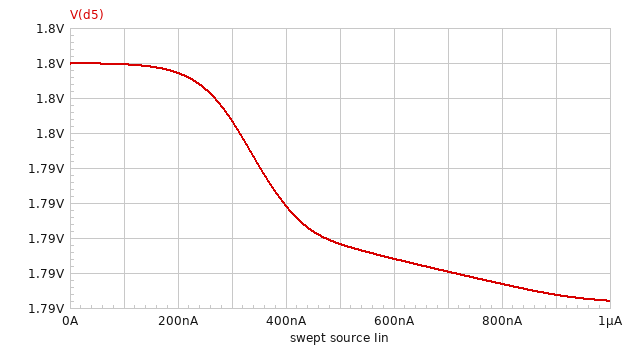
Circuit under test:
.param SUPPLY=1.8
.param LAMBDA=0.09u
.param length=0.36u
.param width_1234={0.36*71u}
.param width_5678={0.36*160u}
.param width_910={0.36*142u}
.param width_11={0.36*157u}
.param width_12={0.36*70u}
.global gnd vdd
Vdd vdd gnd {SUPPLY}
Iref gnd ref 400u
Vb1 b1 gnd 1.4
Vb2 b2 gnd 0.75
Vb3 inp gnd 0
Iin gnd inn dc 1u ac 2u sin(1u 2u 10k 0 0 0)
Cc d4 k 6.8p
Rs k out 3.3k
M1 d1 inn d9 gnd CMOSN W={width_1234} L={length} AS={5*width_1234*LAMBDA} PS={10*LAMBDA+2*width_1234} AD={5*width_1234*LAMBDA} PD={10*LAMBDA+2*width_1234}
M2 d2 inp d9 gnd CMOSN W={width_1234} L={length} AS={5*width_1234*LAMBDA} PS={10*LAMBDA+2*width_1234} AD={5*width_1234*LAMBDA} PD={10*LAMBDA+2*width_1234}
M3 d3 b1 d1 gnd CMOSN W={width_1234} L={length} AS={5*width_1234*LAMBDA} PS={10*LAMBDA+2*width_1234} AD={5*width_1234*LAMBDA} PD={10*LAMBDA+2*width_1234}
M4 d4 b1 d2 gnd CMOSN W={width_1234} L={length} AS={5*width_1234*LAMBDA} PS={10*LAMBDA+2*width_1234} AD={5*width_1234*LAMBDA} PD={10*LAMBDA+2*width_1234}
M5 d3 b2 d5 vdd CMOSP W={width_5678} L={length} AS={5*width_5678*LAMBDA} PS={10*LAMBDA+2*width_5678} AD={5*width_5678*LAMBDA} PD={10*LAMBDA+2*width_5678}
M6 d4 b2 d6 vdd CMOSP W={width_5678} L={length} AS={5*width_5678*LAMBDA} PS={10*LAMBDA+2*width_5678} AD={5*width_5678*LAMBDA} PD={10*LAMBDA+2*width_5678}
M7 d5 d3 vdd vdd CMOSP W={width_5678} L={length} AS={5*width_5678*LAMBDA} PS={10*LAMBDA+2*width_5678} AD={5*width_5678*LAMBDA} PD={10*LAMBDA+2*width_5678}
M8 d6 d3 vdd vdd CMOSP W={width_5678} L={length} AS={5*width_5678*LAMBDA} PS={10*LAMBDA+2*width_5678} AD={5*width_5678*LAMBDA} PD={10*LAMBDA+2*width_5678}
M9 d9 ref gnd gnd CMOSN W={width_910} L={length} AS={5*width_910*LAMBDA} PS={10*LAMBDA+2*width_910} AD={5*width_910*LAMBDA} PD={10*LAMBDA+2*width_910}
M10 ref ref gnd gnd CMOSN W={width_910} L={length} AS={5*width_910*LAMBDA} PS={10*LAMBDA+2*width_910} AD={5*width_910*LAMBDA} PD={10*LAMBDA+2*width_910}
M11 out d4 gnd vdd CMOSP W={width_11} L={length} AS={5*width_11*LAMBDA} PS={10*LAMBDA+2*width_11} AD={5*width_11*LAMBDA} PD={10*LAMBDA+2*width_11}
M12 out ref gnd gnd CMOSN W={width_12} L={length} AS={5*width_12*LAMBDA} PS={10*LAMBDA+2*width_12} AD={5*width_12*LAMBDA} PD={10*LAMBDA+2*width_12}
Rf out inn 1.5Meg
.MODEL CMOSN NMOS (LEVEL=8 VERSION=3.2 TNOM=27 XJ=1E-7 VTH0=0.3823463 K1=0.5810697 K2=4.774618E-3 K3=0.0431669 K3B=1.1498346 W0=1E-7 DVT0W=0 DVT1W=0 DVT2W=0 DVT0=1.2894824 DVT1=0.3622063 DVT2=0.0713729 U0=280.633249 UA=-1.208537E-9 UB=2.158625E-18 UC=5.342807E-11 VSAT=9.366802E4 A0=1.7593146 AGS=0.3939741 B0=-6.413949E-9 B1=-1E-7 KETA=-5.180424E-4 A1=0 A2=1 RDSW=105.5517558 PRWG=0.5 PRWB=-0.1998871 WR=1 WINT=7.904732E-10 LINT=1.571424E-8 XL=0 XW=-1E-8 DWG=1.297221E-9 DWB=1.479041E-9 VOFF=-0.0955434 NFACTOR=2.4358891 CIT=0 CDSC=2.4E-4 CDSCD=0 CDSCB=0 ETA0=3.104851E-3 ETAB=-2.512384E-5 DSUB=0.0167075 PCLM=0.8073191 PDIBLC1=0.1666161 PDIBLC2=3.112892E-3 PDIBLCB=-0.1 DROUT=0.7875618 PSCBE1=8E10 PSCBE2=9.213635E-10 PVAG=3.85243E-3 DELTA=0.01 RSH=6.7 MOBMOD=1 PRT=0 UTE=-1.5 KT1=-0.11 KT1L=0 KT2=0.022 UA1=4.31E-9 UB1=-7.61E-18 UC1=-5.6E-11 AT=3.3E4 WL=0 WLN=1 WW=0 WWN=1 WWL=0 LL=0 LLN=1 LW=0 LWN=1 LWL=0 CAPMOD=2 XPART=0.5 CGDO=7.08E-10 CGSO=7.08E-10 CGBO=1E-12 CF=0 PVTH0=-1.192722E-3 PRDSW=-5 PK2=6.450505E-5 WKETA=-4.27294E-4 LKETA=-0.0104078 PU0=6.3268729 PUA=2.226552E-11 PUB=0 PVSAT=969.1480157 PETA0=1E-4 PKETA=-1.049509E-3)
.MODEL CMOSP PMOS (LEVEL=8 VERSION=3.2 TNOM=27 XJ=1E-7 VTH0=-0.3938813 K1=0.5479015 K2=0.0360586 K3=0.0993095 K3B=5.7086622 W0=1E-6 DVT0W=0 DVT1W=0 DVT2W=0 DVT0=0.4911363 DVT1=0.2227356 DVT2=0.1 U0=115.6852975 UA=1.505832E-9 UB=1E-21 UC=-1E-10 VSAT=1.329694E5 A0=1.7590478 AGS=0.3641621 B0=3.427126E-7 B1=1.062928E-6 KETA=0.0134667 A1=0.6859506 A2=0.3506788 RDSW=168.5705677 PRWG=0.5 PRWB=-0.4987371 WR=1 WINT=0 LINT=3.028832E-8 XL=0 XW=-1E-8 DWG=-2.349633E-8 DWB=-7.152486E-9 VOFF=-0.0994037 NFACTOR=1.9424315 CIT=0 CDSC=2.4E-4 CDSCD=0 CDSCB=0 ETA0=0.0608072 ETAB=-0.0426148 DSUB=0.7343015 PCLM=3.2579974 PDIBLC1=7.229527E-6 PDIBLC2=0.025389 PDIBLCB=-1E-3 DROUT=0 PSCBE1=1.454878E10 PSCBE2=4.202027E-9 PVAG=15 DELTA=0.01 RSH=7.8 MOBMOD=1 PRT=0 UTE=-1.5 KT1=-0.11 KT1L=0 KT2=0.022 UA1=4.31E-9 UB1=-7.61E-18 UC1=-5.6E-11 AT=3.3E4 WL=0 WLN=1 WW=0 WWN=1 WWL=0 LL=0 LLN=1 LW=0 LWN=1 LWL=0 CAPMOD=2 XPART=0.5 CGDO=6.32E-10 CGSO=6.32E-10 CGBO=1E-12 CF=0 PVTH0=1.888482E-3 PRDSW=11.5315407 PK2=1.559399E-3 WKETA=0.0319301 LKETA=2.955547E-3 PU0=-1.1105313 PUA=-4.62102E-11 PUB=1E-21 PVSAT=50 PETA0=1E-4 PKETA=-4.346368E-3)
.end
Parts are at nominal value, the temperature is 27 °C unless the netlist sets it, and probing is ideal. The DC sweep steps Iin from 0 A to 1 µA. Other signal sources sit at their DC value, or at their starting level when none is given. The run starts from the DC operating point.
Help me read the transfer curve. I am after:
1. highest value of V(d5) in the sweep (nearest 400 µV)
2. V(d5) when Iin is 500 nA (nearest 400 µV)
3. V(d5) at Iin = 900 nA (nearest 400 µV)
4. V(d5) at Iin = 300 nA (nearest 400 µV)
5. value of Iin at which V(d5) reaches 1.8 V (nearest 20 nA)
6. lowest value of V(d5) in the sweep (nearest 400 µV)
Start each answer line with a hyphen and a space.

- 1.8000 V
- 1.7896 V
- 1.7868 V
- 1.7968 V
- 320 nA
- 1.7864 V
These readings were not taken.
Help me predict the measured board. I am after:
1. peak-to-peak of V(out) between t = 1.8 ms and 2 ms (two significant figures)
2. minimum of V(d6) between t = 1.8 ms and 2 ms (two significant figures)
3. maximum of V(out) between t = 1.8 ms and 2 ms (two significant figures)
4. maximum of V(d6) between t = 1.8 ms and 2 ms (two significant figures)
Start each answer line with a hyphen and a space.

- 2.3 mV
- 1.8 V
- 1.7 mV
- 1.8 V
